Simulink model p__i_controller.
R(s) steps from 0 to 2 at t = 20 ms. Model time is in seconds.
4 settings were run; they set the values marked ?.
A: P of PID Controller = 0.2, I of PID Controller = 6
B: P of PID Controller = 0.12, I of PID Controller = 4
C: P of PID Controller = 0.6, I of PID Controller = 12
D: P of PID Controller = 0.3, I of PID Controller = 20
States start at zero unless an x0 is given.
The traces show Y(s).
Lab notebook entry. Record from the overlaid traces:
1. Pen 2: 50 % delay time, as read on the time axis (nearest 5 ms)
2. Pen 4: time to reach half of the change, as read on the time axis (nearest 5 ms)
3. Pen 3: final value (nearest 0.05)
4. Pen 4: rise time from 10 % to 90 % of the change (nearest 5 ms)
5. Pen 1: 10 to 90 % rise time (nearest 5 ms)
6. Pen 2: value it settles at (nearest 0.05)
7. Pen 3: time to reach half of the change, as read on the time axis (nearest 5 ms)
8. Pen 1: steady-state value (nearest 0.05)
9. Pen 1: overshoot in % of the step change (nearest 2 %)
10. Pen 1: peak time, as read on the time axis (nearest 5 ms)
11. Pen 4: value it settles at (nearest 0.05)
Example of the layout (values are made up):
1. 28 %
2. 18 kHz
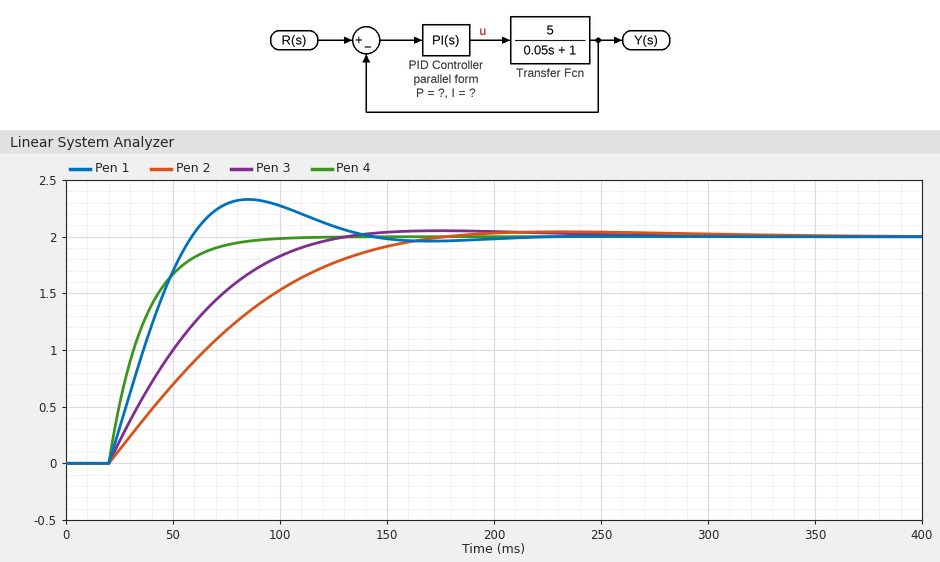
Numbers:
1. 65 ms
2. 30 ms
3. 2.00
4. 35 ms
5. 30 ms
6. 2.00
7. 50 ms
8. 2.00
9. 16 %
10. 85 ms
11. 2.00
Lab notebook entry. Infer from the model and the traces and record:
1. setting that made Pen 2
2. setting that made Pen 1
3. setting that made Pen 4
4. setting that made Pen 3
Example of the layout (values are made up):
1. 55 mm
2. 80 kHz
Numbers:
1. B
2. D
3. C
4. A
